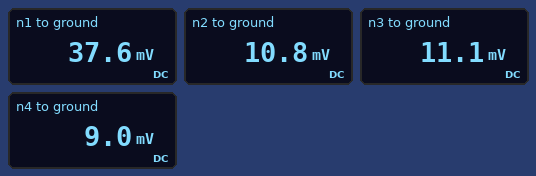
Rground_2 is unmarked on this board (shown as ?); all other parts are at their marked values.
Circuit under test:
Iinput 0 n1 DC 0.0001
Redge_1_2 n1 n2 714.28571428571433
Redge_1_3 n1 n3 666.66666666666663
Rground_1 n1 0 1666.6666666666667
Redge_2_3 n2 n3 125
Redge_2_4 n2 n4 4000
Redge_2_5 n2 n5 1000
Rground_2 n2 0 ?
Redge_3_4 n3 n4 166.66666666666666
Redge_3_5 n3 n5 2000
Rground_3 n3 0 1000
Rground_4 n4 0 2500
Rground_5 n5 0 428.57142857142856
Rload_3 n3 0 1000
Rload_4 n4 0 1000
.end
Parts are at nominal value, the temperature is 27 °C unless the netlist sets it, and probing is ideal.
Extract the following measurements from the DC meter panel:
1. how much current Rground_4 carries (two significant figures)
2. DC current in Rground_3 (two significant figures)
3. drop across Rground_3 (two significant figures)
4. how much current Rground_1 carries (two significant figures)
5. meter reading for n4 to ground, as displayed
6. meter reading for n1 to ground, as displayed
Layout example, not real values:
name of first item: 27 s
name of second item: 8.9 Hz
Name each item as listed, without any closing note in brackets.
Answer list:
how much current Rground_4 carries: 3.6 µA
DC current in Rground_3: 11 µA
drop across Rground_3: 11 mV
how much current Rground_1 carries: 23 µA
meter reading for n4 to ground, as displayed: 9.0 mV
meter reading for n1 to ground, as displayed: 37.6 mV
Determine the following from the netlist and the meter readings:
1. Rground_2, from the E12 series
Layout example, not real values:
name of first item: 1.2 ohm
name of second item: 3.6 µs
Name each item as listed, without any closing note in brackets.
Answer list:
Rground_2, from the E12 series: 330 Ω
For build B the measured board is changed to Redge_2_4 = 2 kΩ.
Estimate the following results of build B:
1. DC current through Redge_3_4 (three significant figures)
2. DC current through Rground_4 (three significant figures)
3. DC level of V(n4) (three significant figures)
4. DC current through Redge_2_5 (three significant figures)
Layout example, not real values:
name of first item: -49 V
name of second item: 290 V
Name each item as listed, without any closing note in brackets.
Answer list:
DC current through Redge_3_4: 11.9 µA
DC current through Rground_4: 3.64 µA
DC level of V(n4): 9.09 mV
DC current through Redge_2_5: 6.52 µA
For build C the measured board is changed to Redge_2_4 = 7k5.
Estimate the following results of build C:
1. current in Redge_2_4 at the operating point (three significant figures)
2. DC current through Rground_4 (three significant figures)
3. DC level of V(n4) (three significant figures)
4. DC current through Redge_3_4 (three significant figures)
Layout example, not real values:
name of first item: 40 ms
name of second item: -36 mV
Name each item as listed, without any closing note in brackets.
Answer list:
current in Redge_2_4 at the operating point: 241 nA
DC current through Rground_4: 3.60 µA
DC level of V(n4): 9.00 mV
DC current through Redge_3_4: 12.4 µA
